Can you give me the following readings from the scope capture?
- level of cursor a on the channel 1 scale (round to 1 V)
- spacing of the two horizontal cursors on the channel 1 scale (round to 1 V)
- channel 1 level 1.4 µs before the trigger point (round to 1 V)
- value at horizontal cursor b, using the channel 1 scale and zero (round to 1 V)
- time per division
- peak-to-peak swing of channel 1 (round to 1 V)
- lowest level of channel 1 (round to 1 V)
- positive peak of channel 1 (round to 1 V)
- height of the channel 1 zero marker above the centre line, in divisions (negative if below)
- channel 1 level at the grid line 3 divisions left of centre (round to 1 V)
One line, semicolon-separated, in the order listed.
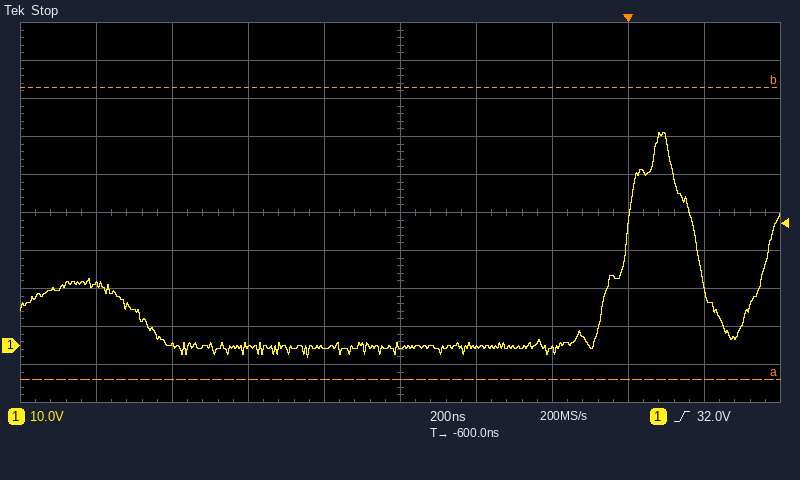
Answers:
-9 V; 77 V; 16 V; 68 V; 200 ns; 59 V; -3 V; 56 V; -3.5 div; 0 V
